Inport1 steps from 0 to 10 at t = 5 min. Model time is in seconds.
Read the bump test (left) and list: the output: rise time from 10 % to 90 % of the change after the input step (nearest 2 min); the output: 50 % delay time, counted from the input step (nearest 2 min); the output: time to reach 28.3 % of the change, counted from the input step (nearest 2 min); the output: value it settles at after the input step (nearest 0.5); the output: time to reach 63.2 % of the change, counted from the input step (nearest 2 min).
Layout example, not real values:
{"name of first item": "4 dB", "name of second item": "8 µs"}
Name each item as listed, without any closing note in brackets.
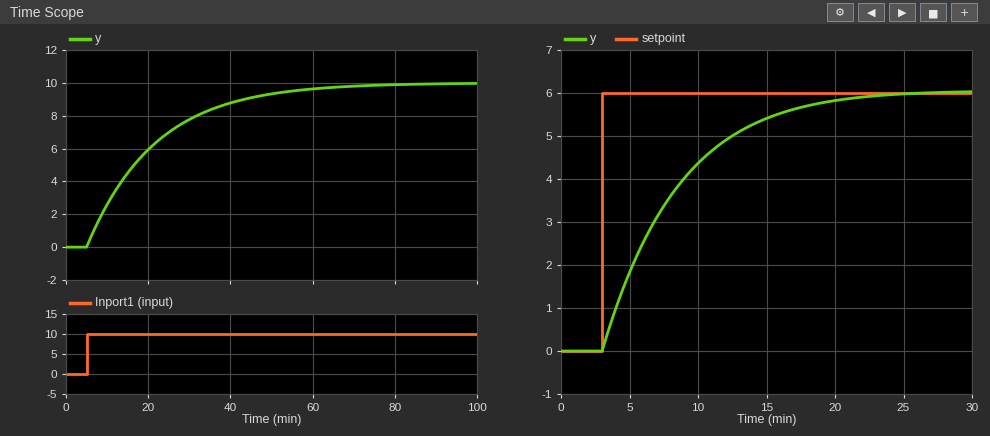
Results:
{"the output: rise time from 10 % to 90 % of the change after the input step": "36 min", "the output: 50 % delay time, counted from the input step": "12 min", "the output: time to reach 28.3 % of the change, counted from the input step": "6 min", "the output: value it settles at after the input step": "10.0", "the output: time to reach 63.2 % of the change, counted from the input step": "16 min"}
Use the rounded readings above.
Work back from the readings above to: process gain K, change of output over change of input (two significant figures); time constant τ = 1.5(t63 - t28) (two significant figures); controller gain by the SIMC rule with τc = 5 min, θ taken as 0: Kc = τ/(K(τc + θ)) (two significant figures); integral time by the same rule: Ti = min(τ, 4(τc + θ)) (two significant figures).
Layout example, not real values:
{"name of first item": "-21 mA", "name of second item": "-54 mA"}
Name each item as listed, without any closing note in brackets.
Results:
{"process gain K, change of output over change of input": "1.0", "time constant τ = 1.5(t63 - t28)": "15 min", "controller gain by the SIMC rule with τc = 5 min, θ taken as 0: Kc = τ/(K(τc + θ))": "3.0", "integral time by the same rule: Ti = min(τ, 4(τc + θ))": "15 min"}
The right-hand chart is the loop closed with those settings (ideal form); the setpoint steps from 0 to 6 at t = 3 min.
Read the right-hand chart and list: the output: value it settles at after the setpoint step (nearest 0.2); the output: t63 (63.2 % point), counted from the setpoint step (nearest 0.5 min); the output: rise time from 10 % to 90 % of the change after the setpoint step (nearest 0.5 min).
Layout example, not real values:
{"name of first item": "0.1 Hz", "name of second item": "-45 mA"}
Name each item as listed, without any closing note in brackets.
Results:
{"the output: value it settles at after the setpoint step": "6.0", "the output: t63 (63.2 % point), counted from the setpoint step": "5.5 min", "the output: rise time from 10 % to 90 % of the change after the setpoint step": "11.5 min"}
